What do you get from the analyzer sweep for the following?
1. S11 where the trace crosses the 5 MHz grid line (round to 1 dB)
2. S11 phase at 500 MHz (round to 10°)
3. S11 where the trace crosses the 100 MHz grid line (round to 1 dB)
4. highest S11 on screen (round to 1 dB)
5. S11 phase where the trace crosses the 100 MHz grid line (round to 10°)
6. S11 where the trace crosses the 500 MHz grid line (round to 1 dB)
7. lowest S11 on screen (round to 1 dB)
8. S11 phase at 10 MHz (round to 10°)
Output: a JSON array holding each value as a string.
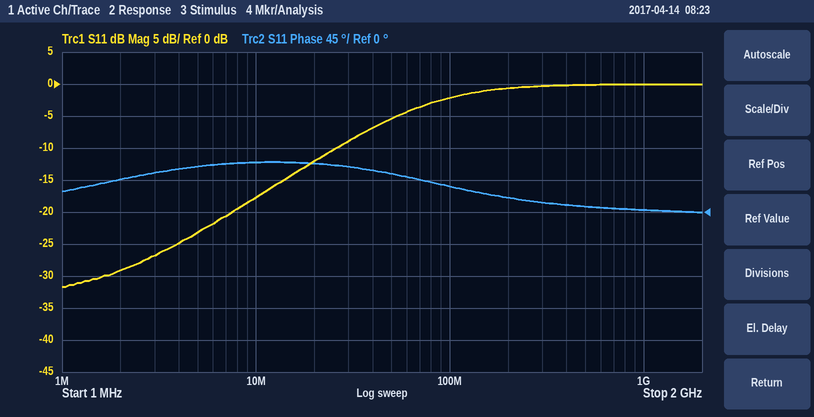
["-23 dB", "10°", "-2 dB", "0 dB", "40°", "0 dB", "-32 dB", "70°"]
